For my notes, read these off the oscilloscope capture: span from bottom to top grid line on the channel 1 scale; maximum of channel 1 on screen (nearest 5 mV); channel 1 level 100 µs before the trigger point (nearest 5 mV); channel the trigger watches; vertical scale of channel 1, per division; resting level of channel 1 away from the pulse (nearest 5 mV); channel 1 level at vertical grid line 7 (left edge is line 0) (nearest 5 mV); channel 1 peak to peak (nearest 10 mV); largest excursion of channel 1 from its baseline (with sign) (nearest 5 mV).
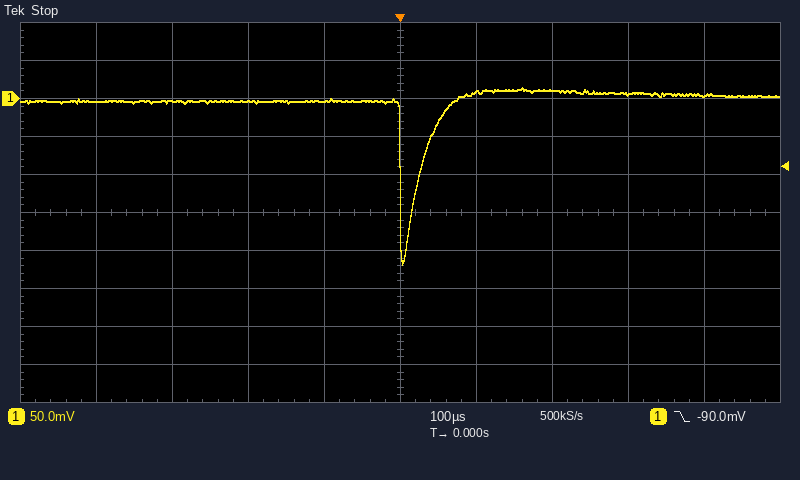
500 mV
15 mV
-5 mV
channel 1
50 mV
-5 mV
10 mV
230 mV
-215 mV
